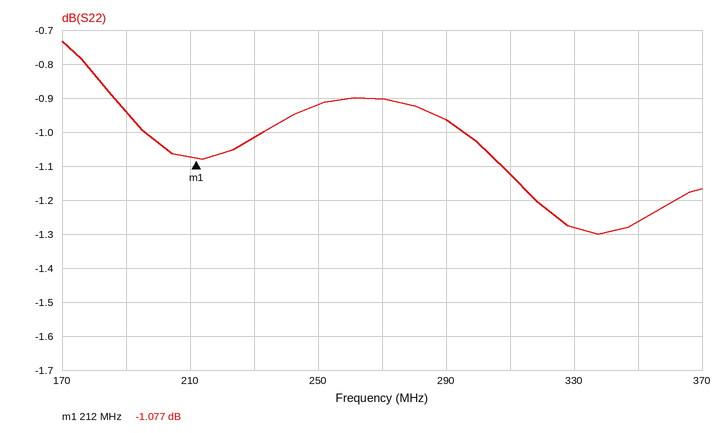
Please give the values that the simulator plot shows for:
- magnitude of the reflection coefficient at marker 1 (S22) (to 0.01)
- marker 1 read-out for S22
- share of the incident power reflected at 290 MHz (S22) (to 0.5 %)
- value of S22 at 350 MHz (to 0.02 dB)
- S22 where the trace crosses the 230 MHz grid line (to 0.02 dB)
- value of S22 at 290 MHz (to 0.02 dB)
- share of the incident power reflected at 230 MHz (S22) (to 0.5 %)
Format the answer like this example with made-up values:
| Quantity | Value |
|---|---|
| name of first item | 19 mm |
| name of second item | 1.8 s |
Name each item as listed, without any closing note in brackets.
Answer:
| Quantity | Value |
|---|---|
| magnitude of the reflection coefficient at marker 1 (S22) | 0.88 |
| marker 1 read-out for S22 | -1.077 dB |
| share of the incident power reflected at 290 MHz (S22) | 80.0 % |
| value of S22 at 350 MHz | -1.26 dB |
| S22 where the trace crosses the 230 MHz grid line | -1.02 dB |
| value of S22 at 290 MHz | -0.96 dB |
| share of the incident power reflected at 230 MHz (S22) | 79.0 % |
